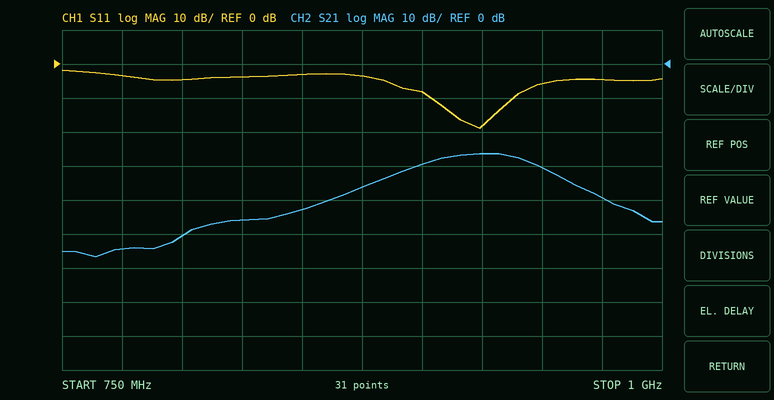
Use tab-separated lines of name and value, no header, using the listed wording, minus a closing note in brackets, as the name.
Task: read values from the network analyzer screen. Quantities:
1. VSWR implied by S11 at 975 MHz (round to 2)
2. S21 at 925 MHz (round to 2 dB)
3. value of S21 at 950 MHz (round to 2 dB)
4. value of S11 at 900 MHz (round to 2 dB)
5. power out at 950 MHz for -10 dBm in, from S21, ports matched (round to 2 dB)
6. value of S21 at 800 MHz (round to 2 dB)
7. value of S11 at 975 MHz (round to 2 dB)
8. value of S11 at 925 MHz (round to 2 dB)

VSWR implied by S11 at 975 MHz	4
S21 at 925 MHz	-26 dB
value of S21 at 950 MHz	-30 dB
value of S11 at 900 MHz	-8 dB
power out at 950 MHz for -10 dBm in, from S21, ports matched	-40 dBm
value of S21 at 800 MHz	-50 dB
value of S11 at 975 MHz	-4 dB
value of S11 at 925 MHz	-18 dB
